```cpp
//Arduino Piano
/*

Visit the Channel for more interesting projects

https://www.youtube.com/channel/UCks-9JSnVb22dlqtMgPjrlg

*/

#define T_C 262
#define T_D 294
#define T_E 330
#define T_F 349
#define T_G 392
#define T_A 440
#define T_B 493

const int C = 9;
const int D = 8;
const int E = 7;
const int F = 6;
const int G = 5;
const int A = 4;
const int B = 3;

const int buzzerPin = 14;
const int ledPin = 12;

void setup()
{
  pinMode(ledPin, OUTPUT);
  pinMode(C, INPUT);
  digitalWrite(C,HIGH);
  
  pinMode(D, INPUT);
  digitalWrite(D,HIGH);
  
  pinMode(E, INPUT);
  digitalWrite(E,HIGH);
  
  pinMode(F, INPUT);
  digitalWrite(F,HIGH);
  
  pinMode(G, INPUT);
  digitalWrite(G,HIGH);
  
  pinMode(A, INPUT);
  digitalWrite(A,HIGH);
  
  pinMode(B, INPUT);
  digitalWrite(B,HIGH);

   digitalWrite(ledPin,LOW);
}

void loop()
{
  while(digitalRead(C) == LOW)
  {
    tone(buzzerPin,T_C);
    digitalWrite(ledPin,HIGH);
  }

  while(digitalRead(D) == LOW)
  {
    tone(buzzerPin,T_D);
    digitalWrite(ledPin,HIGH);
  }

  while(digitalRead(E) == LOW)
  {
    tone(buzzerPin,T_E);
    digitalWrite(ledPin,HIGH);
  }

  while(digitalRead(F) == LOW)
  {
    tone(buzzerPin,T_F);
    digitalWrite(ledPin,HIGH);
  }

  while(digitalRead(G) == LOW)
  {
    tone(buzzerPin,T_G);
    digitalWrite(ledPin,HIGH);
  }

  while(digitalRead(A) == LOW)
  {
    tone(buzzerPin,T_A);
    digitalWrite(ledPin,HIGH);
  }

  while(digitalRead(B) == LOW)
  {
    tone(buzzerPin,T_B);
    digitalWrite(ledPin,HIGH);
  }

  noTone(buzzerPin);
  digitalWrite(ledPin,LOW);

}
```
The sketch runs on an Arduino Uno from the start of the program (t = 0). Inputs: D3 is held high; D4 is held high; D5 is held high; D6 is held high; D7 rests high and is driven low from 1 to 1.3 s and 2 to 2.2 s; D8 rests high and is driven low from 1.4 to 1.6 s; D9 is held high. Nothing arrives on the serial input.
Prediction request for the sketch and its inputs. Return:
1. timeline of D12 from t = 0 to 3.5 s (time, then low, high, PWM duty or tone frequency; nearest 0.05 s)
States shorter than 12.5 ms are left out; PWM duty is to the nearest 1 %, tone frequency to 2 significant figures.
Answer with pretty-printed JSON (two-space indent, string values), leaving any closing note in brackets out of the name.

{
  "timeline of D12 from t = 0 to 3.5 s": "0 s low; 1 s high; 1.3 s low; 1.4 s high; 1.6 s low; 2 s high; 2.2 s low"
}
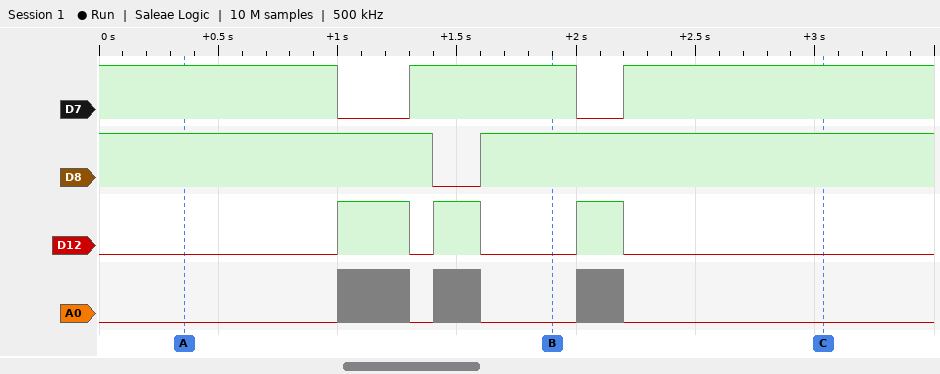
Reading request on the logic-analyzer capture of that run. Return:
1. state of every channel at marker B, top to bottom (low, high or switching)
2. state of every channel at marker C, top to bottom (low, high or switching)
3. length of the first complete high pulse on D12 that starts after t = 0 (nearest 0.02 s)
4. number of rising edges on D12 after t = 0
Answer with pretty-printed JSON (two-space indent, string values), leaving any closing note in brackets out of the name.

{
  "state of every channel at marker B, top to bottom": "D7 high, D8 high, D12 low, A0 low",
  "state of every channel at marker C, top to bottom": "D7 high, D8 high, D12 low, A0 low",
  "length of the first complete high pulse on D12 that starts after t = 0": "0.30 s",
  "number of rising edges on D12 after t = 0": "3"
}
